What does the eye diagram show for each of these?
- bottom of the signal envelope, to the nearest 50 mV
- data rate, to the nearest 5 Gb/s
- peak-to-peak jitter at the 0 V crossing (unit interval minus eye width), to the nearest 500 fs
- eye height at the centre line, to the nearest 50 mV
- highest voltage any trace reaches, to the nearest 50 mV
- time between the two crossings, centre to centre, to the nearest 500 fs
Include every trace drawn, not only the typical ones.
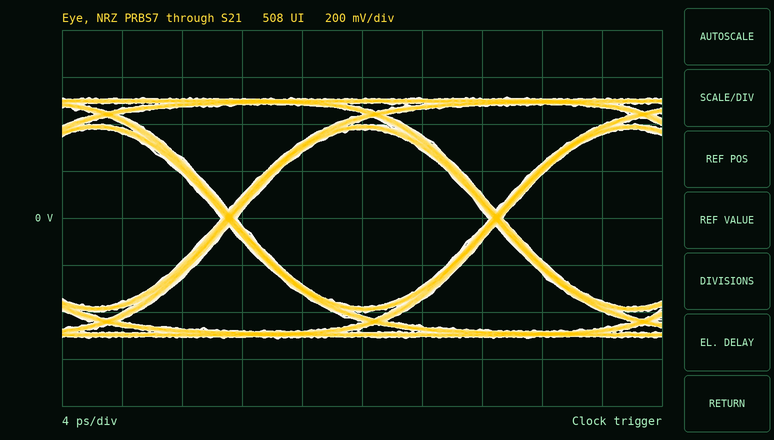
-500 mV
55 Gb/s
1.0 ps
750 mV
500 mV
18.0 ps
